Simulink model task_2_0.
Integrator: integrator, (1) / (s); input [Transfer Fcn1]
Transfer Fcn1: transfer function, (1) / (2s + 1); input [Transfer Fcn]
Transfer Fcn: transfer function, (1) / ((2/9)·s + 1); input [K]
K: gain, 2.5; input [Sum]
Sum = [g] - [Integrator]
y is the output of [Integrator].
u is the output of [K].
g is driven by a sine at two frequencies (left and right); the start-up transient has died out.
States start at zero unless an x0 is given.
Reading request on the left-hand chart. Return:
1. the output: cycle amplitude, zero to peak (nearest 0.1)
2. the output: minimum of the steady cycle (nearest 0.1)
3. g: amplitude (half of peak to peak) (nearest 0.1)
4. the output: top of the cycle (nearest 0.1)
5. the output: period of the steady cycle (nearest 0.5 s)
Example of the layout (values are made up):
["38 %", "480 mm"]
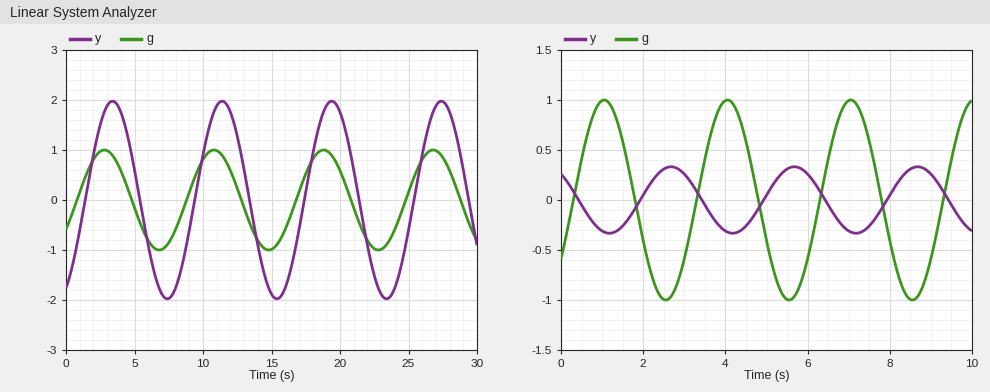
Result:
["2.0", "-2.0", "1.0", "2.0", "8.0 s"]
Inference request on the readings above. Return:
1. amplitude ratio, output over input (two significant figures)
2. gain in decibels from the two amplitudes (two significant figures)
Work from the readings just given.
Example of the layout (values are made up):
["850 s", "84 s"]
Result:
["2.0", "6.0 dB"]
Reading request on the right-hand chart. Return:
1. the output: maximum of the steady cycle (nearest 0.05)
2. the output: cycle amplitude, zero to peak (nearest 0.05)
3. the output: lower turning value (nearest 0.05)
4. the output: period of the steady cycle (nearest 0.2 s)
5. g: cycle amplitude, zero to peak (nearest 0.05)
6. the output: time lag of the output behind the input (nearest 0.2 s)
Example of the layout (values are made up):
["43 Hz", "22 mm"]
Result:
["0.35", "0.35", "-0.35", "3.0 s", "1.00", "1.6 s"]
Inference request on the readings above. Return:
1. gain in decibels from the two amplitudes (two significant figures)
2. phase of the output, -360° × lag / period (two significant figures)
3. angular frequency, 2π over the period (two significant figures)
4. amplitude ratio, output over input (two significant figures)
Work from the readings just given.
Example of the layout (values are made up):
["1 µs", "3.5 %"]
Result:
["-9.1 dB", "-190°", "2.1 rad/s", "0.35"]
